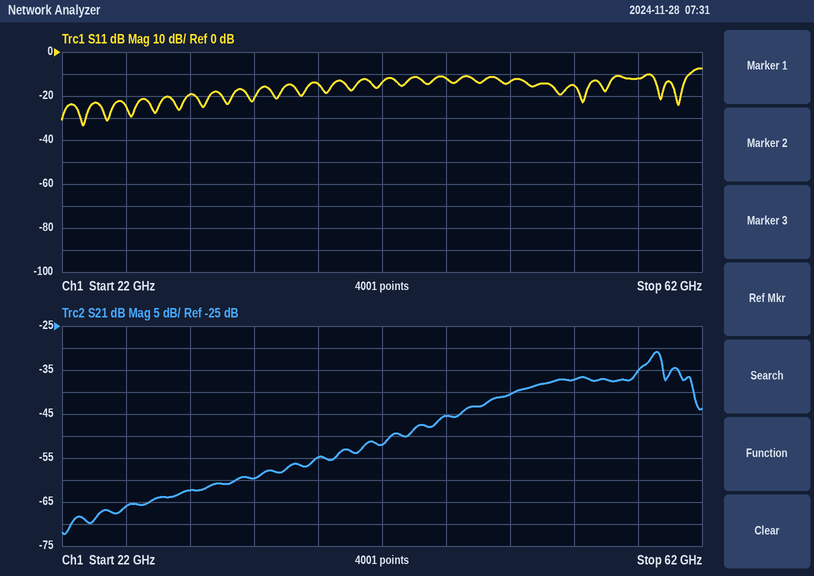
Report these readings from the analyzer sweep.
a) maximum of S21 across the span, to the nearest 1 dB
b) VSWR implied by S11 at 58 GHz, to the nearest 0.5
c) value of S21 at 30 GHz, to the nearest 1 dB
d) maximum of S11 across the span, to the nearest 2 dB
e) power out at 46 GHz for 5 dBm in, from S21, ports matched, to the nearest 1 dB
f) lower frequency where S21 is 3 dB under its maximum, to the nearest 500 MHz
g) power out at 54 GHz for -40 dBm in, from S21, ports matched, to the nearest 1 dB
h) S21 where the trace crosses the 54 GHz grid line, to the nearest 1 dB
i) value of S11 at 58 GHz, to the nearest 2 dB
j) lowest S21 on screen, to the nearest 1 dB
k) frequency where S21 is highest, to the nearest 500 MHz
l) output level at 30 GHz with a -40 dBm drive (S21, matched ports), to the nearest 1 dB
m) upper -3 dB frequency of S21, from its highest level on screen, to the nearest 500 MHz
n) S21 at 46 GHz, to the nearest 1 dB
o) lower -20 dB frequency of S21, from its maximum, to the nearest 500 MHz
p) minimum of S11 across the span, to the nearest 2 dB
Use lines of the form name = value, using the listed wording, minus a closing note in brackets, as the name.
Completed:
maximum of S21 across the span, to the nearest 1 dB = -31 dB
VSWR implied by S11 at 58 GHz, to the nearest 0.5 = 1.5
value of S21 at 30 GHz, to the nearest 1 dB = -62 dB
maximum of S11 across the span, to the nearest 2 dB = -8 dB
power out at 46 GHz for 5 dBm in, from S21, ports matched, to the nearest 1 dB = -40 dBm
lower frequency where S21 is 3 dB under its maximum, to the nearest 500 MHz = 58.5 GHz
power out at 54 GHz for -40 dBm in, from S21, ports matched, to the nearest 1 dB = -77 dBm
S21 where the trace crosses the 54 GHz grid line, to the nearest 1 dB = -37 dB
value of S11 at 58 GHz, to the nearest 2 dB = -12 dB
lowest S21 on screen, to the nearest 1 dB = -72 dB
frequency where S21 is highest, to the nearest 500 MHz = 59.0 GHz
output level at 30 GHz with a -40 dBm drive (S21, matched ports), to the nearest 1 dB = -102 dBm
upper -3 dB frequency of S21, from its highest level on screen, to the nearest 500 MHz = 59.5 GHz
S21 at 46 GHz, to the nearest 1 dB = -45 dB
lower -20 dB frequency of S21, from its maximum, to the nearest 500 MHz = 42.5 GHz
minimum of S11 across the span, to the nearest 2 dB = -34 dB
